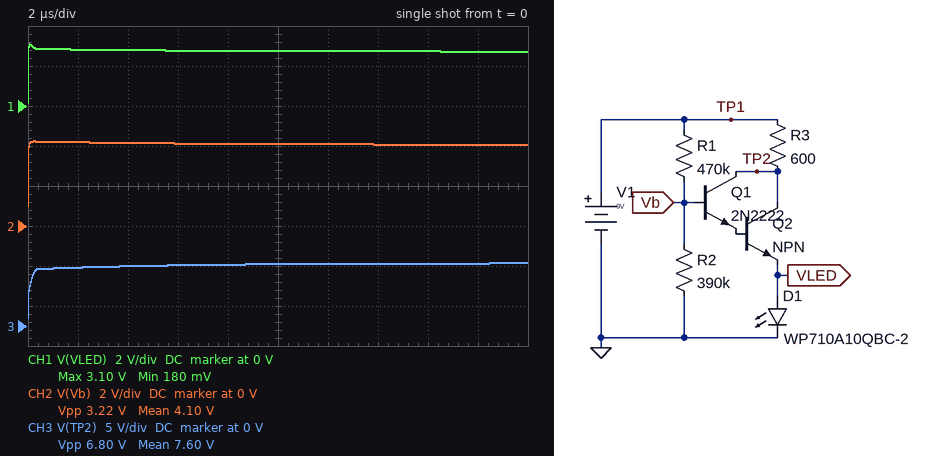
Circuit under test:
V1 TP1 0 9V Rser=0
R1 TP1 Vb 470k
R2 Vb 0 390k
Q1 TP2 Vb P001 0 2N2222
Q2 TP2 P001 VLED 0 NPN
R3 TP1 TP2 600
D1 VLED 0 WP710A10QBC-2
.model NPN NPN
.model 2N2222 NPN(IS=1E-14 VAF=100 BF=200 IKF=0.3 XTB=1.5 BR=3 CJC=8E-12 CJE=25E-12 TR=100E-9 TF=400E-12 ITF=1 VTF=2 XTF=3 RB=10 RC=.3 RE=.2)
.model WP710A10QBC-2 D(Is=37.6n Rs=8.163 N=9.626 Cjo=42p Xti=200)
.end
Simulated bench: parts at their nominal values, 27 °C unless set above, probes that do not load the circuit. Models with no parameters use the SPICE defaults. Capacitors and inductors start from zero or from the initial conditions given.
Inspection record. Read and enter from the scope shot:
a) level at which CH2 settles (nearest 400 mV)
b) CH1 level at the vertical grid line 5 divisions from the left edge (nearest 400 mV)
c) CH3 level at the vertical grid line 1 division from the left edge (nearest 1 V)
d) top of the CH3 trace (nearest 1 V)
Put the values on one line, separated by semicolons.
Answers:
4.0 V; 2.8 V; 7 V; 8 V
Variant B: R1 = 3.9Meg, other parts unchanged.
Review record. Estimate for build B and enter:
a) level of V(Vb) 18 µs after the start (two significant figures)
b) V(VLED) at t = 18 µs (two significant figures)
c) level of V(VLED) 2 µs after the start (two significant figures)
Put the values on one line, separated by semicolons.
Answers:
840 mV; 920 mV; 1.9 V
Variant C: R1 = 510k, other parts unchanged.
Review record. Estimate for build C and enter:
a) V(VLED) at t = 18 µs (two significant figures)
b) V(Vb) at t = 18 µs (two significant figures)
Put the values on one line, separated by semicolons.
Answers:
2.6 V; 3.9 V
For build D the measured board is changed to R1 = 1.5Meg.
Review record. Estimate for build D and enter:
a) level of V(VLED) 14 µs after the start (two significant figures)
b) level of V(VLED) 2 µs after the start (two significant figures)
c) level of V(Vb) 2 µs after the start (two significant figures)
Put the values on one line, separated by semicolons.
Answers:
1.0 V; 2.2 V; 3.4 V
